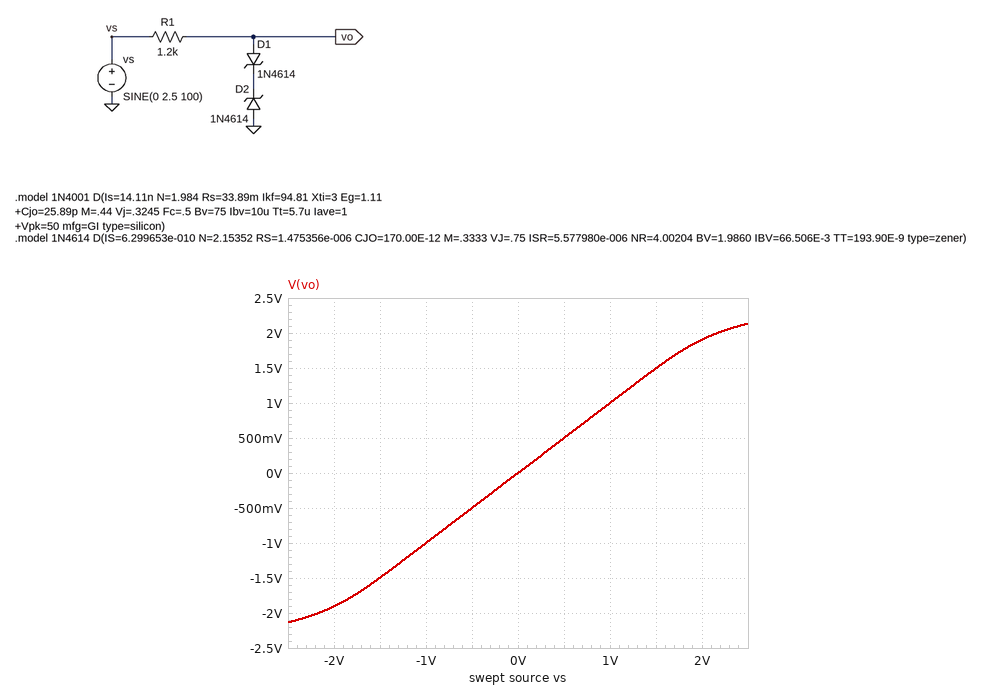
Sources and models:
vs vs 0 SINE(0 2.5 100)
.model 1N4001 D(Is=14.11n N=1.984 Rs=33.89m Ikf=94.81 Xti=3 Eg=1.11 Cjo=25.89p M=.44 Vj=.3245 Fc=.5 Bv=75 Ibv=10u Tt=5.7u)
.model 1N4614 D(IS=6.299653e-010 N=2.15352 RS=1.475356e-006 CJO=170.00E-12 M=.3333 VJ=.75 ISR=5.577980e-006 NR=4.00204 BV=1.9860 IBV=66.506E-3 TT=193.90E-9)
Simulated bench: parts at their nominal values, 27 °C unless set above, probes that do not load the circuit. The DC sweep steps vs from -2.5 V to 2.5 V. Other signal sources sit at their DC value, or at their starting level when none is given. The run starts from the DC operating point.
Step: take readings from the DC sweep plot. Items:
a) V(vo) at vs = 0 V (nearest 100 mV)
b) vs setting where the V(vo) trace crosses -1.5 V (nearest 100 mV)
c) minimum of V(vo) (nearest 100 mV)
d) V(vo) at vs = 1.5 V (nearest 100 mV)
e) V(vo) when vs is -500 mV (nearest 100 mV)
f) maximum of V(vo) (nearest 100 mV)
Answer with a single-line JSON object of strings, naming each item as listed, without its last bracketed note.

{"V(vo) at vs = 0 V": "0 V", "vs setting where the V(vo) trace crosses -1.5 V": "-1.5 V", "minimum of V(vo)": "-2.1 V", "V(vo) at vs = 1.5 V": "1.5 V", "V(vo) when vs is -500 mV": "-500 mV", "maximum of V(vo)": "2.1 V"}
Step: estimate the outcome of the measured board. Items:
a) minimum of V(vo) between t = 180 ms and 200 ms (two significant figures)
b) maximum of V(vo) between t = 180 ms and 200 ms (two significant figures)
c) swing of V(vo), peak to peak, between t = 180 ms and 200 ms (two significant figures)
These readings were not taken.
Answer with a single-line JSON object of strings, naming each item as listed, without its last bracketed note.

{"minimum of V(vo) between t = 180 ms and 200 ms": "-2.1 V", "maximum of V(vo) between t = 180 ms and 200 ms": "2.1 V", "swing of V(vo), peak to peak, between t = 180 ms and 200 ms": "4.3 V"}
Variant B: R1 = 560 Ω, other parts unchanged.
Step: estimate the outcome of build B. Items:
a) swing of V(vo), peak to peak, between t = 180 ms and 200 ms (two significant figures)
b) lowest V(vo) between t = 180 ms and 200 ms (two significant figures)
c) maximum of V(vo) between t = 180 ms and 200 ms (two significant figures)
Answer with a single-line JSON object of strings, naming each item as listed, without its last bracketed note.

{"swing of V(vo), peak to peak, between t = 180 ms and 200 ms": "4.4 V", "lowest V(vo) between t = 180 ms and 200 ms": "-2.2 V", "maximum of V(vo) between t = 180 ms and 200 ms": "2.2 V"}
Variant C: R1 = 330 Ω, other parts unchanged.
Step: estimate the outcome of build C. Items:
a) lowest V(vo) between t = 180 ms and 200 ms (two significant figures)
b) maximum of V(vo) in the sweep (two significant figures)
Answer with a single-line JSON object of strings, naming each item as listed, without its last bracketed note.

{"lowest V(vo) between t = 180 ms and 200 ms": "-2.3 V", "maximum of V(vo) in the sweep": "2.3 V"}
